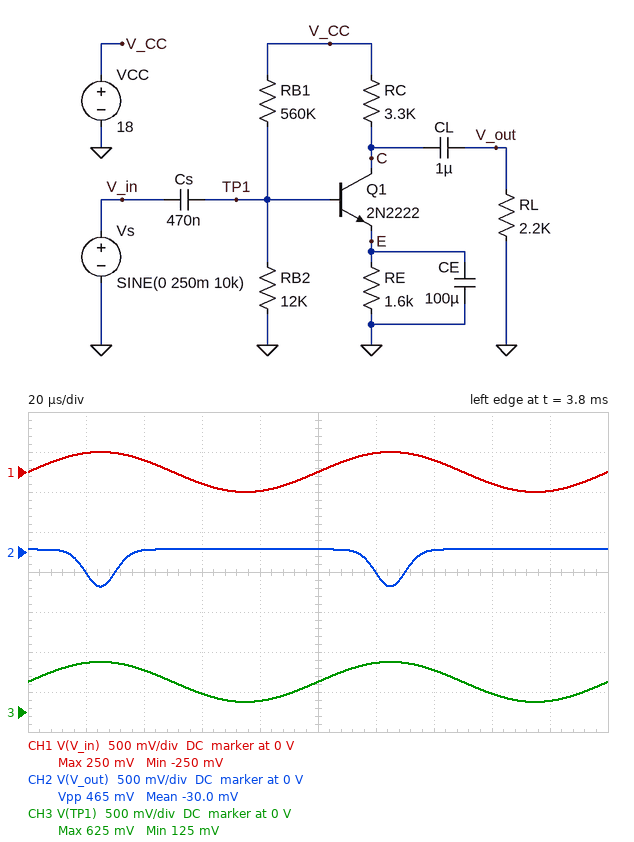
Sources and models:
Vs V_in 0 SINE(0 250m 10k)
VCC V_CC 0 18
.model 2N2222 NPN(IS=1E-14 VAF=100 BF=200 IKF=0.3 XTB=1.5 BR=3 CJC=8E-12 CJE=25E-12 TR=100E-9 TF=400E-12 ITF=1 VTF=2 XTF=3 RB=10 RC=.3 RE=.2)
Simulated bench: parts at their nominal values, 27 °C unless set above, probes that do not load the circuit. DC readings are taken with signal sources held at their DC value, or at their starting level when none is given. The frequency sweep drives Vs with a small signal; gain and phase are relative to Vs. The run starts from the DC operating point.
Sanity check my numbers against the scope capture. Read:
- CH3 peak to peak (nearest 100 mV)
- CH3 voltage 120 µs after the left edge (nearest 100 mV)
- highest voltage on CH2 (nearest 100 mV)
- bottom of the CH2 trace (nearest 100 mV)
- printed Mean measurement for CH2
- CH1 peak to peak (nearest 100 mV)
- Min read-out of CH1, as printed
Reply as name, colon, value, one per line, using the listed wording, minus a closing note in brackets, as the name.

CH3 peak to peak: 500 mV
CH3 voltage 120 µs after the left edge: 600 mV
highest voltage on CH2: 0 V
bottom of the CH2 trace: -400 mV
printed Mean measurement for CH2: -30.0 mV
CH1 peak to peak: 500 mV
Min read-out of CH1, as printed: -250 mV
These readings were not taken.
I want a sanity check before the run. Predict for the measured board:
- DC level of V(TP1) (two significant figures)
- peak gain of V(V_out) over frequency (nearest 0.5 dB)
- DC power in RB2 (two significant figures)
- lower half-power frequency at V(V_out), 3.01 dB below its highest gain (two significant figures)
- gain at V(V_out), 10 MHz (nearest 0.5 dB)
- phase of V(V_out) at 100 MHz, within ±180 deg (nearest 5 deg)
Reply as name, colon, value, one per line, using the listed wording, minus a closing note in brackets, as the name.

DC level of V(TP1): 380 mV
peak gain of V(V_out) over frequency: -1.0 dB
DC power in RB2: 12 µW
lower half-power frequency at V(V_out), 3.01 dB below its highest gain: 37 MHz
gain at V(V_out), 10 MHz: -13.0 dB
phase of V(V_out) at 100 MHz, within ±180 deg: 10 deg
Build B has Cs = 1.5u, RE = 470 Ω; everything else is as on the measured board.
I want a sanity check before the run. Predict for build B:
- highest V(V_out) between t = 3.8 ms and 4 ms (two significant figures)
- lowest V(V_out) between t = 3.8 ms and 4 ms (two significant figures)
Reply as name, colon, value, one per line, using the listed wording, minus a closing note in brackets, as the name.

highest V(V_out) between t = 3.8 ms and 4 ms: 34 mV
lowest V(V_out) between t = 3.8 ms and 4 ms: -450 mV
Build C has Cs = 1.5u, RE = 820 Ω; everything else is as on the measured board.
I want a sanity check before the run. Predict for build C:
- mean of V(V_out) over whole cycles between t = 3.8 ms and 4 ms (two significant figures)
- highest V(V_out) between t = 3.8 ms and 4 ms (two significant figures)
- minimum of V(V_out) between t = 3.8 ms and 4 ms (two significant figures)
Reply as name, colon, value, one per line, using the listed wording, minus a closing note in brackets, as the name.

mean of V(V_out) over whole cycles between t = 3.8 ms and 4 ms: -29 mV
highest V(V_out) between t = 3.8 ms and 4 ms: 34 mV
minimum of V(V_out) between t = 3.8 ms and 4 ms: -450 mV
